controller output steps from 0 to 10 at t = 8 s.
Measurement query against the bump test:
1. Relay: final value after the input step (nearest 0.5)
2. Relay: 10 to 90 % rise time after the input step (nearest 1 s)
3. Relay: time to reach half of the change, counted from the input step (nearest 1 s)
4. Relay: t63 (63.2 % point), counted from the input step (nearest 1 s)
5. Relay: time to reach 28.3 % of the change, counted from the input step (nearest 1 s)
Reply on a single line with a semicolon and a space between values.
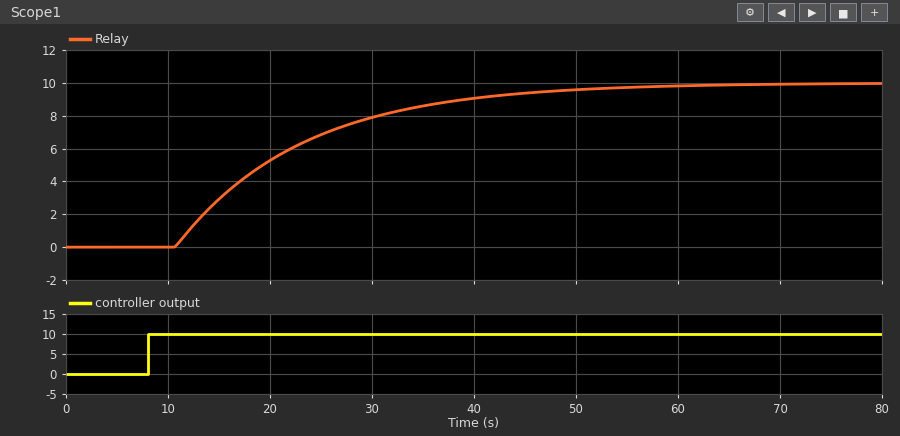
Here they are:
10.0; 27 s; 11 s; 15 s; 7 s
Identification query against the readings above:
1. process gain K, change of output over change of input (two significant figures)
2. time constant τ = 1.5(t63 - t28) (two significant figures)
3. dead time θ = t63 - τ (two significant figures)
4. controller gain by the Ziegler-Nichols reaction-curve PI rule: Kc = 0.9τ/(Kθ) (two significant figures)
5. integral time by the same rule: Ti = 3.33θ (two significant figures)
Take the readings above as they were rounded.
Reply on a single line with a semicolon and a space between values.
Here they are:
1.0; 12 s; 3.0 s; 3.6; 10.0 s
